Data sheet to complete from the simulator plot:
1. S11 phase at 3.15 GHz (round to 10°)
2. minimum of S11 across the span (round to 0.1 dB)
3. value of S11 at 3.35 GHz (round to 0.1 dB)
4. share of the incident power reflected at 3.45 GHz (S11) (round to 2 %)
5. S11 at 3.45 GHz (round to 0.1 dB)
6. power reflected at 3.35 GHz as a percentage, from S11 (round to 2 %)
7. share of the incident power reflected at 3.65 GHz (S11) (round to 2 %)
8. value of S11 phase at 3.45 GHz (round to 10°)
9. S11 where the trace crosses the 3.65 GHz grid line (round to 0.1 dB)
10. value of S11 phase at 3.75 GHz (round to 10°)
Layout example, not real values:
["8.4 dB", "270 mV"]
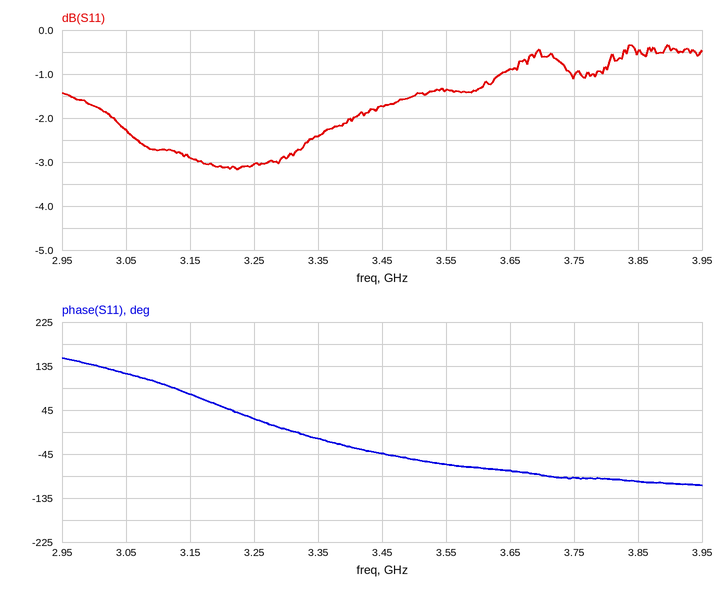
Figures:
["80°", "-3.2 dB", "-2.4 dB", "68 %", "-1.7 dB", "58 %", "82 %", "-40°", "-0.9 dB", "-90°"]
